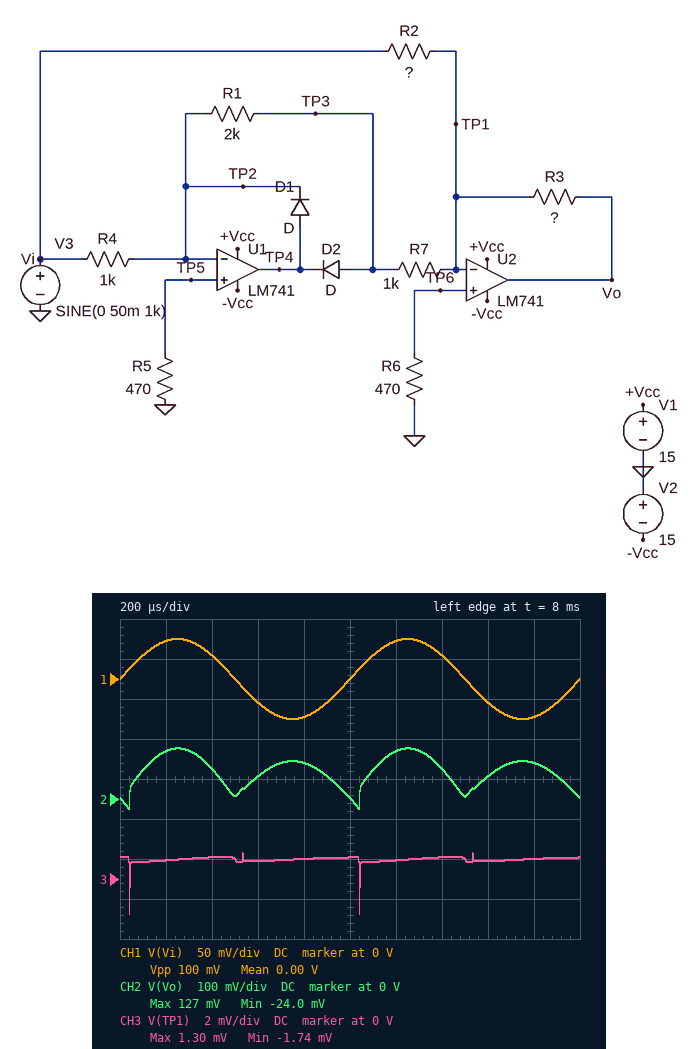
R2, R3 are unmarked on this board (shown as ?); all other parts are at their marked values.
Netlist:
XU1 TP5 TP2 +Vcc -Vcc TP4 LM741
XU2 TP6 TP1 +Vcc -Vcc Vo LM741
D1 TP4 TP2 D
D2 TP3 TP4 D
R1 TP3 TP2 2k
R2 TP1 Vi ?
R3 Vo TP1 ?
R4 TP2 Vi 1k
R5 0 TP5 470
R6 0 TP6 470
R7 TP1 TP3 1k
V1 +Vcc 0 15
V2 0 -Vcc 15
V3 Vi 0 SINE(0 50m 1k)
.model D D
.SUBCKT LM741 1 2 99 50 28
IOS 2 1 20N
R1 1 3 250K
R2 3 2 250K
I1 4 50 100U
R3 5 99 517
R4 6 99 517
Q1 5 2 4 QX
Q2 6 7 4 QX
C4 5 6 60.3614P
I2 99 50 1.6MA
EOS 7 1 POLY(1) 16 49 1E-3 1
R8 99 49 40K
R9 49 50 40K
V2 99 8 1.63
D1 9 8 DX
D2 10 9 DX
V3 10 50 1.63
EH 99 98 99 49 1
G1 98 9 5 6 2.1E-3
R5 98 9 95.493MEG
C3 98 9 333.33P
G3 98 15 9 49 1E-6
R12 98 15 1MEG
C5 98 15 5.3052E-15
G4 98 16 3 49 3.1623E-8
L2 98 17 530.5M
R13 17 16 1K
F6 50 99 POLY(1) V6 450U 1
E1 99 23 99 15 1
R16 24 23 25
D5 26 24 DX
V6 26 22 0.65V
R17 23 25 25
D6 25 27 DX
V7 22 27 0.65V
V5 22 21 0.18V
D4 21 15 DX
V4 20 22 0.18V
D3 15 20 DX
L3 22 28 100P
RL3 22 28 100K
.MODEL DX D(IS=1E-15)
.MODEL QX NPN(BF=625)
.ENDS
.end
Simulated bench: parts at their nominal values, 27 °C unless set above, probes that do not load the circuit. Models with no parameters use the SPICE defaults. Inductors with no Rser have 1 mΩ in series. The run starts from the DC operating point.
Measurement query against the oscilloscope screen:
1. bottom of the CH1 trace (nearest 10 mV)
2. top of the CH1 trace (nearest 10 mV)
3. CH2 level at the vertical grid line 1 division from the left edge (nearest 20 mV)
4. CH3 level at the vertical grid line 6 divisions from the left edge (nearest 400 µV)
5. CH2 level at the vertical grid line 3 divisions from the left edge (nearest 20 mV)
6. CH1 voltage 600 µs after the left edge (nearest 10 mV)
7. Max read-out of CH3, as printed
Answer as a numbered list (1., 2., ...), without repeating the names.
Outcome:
1. -50 mV
2. 50 mV
3. 120 mV
4. 800 µV
5. 60 mV
6. -30 mV
7. 1.30 mV
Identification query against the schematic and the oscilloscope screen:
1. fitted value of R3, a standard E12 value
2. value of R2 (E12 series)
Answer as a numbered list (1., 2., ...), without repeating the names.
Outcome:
1. 2.2 kΩ
2. 1.2 kΩ
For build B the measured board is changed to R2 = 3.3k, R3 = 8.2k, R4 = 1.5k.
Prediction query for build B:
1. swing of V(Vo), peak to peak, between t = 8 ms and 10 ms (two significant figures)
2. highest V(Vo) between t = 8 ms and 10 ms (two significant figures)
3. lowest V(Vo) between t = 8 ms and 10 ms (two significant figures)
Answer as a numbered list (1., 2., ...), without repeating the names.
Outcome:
1. 460 mV
2. 410 mV
3. -46 mV
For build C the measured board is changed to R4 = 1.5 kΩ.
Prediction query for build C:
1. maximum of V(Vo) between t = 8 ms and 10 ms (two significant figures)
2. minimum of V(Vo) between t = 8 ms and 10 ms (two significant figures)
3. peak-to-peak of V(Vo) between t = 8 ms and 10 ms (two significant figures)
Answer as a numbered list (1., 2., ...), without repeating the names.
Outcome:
1. 95 mV
2. -25 mV
3. 120 mV
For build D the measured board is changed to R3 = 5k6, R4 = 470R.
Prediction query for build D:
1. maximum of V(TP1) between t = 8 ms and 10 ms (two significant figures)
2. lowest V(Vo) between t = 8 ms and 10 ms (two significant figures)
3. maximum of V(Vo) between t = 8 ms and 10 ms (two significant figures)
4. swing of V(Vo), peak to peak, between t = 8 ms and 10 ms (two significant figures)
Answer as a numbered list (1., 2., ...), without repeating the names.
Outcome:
1. 1.9 mV
2. -61 mV
3. 940 mV
4. 1.0 V
